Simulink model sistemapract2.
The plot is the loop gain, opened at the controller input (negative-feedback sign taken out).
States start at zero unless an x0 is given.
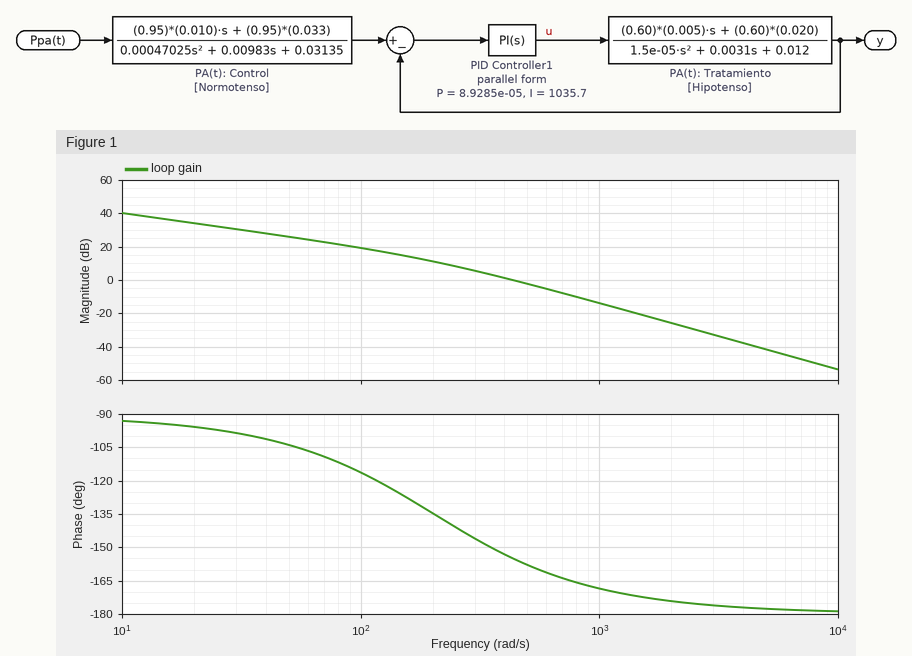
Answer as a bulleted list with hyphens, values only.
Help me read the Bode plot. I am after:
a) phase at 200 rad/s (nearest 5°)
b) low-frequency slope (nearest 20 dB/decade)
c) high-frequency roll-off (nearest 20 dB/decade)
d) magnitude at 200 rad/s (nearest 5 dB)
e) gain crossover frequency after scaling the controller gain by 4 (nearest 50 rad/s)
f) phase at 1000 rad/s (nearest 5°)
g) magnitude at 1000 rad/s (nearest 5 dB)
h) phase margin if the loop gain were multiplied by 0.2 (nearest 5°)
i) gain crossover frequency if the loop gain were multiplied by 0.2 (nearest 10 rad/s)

- -135°
- -20 dB/decade
- -40 dB/decade
- 10 dB
- 900 rad/s
- -170°
- -15 dB
- 50°
- 160 rad/s
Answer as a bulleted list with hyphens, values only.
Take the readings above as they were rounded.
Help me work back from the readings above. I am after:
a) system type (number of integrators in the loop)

- 1
